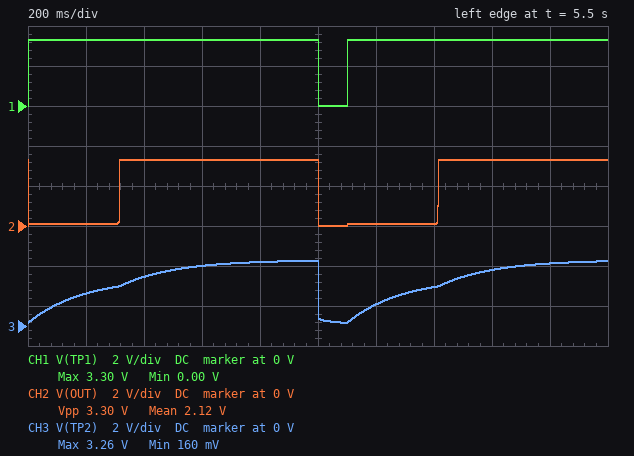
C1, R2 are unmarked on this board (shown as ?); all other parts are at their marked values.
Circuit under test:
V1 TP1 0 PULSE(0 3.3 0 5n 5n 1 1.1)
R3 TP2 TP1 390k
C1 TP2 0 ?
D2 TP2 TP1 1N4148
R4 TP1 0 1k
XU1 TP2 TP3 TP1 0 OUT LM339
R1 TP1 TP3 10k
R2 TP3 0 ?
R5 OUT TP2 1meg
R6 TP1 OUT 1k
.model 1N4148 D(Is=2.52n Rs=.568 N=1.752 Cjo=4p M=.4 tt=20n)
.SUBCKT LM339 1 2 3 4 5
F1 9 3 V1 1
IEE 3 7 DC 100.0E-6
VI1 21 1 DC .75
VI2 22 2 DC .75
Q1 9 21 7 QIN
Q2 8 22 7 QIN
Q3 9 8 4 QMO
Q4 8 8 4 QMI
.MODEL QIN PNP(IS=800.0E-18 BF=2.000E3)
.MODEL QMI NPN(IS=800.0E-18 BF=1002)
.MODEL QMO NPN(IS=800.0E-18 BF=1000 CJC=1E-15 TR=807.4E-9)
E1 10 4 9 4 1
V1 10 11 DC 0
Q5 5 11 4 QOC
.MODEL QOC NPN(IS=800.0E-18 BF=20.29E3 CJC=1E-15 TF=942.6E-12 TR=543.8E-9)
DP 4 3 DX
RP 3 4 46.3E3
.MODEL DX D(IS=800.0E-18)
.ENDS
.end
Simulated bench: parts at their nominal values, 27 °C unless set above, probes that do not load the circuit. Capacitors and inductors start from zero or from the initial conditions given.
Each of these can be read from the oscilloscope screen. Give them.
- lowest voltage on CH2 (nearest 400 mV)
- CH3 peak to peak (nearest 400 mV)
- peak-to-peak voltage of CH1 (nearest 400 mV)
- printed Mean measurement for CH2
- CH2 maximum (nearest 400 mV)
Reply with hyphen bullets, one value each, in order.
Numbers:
- 0 V
- 3.2 V
- 3.2 V
- 2.12 V
- 3.2 V
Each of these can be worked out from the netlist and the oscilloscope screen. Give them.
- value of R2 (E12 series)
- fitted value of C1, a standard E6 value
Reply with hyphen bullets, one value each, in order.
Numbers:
- 15 kΩ
- 680 nF
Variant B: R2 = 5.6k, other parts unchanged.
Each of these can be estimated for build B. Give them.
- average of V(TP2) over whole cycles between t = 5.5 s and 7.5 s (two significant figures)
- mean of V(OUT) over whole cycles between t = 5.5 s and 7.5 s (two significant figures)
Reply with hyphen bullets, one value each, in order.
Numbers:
- 2.4 V
- 2.7 V
